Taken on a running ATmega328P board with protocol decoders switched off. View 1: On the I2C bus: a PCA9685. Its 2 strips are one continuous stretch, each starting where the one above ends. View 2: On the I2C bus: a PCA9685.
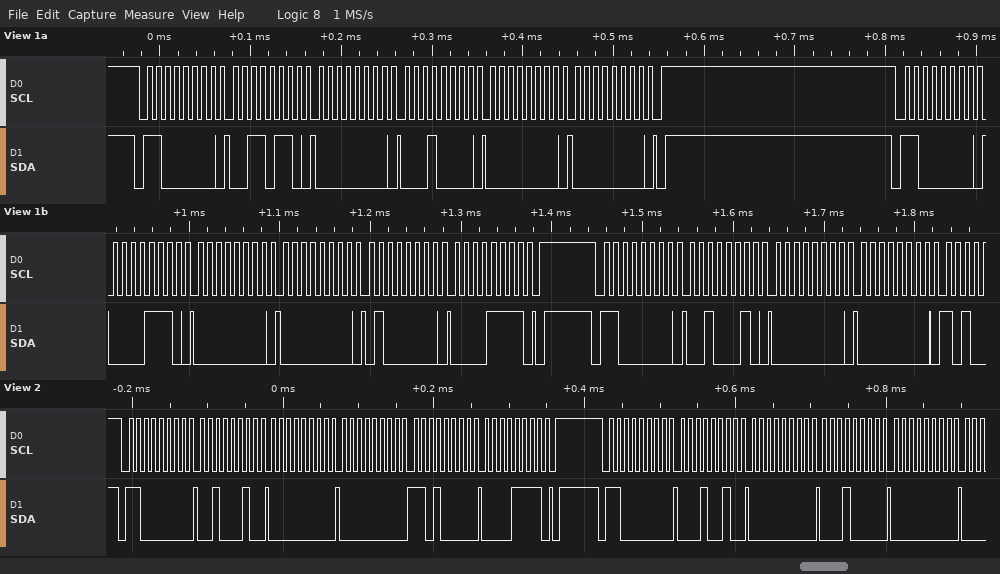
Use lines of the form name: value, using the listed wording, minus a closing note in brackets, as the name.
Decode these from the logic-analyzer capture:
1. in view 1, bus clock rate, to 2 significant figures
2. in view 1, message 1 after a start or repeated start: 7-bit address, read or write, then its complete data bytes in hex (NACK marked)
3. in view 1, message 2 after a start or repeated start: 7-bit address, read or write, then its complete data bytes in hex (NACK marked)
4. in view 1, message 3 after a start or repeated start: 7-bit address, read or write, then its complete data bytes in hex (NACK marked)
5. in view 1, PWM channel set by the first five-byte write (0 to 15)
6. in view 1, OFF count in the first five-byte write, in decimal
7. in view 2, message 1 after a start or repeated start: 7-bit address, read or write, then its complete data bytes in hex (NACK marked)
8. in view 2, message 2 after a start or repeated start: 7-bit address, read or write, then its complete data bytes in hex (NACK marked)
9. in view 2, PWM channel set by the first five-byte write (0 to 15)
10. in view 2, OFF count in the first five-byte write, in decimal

in view 1, bus clock rate, to 2 significant figures: 100 kHz
in view 1, message 1 after a start or repeated start: 7-bit address, read or write, then its complete data bytes in hex: 0x60 write: 36 00 10 00 00
in view 1, message 2 after a start or repeated start: 7-bit address, read or write, then its complete data bytes in hex: 0x60 write: 0E 00 00 40 0F
in view 1, message 3 after a start or repeated start: 7-bit address, read or write, then its complete data bytes in hex: 0x60 write: 22 00 00
in view 1, PWM channel set by the first five-byte write: 12
in view 1, OFF count in the first five-byte write, in decimal: 0
in view 2, message 1 after a start or repeated start: 7-bit address, read or write, then its complete data bytes in hex: 0x60 write: 22 00 00 D0 0F
in view 2, message 2 after a start or repeated start: 7-bit address, read or write, then its complete data bytes in hex: 0x60 write: 12 00 10 00
in view 2, PWM channel set by the first five-byte write: 7
in view 2, OFF count in the first five-byte write, in decimal: 4048
